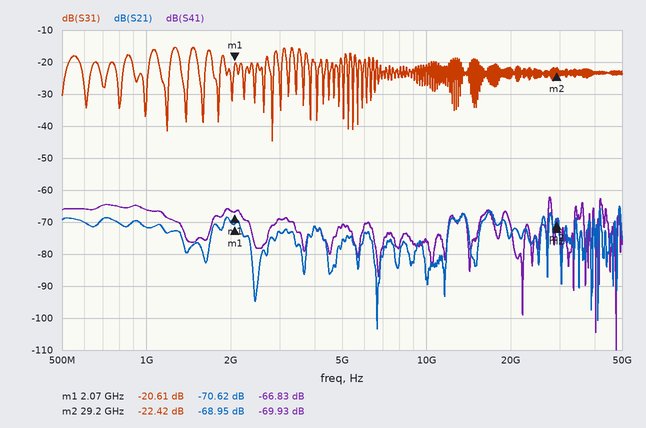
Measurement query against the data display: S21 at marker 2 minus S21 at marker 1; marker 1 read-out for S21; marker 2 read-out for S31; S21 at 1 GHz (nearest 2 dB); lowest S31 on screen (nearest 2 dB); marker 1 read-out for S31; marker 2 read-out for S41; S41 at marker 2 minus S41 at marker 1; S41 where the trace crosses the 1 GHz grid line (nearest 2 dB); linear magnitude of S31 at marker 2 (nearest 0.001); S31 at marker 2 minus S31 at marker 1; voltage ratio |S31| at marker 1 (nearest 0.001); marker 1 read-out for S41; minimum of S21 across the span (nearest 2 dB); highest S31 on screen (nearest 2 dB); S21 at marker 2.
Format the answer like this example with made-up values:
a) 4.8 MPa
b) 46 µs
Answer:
a) 1.67 dB
b) -70.62 dB
c) -22.42 dB
d) -72 dB
e) -44 dB
f) -20.61 dB
g) -69.93 dB
h) -3.10 dB
i) -66 dB
j) 0.076
k) -1.81 dB
l) 0.093
m) -66.83 dB
n) -104 dB
o) -16 dB
p) -68.95 dB
